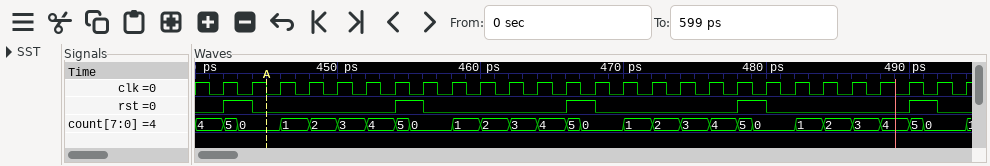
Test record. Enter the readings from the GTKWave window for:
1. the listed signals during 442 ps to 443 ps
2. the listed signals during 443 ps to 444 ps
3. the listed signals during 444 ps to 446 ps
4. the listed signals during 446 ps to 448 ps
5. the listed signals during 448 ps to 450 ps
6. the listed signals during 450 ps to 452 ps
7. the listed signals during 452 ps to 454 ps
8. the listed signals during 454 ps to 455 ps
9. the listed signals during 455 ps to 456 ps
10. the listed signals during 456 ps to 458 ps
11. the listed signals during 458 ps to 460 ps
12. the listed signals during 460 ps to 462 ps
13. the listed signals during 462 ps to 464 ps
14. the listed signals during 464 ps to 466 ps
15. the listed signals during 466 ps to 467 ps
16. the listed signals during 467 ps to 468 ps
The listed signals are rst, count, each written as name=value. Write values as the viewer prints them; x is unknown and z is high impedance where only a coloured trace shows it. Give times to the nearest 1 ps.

rst=1, count=5
rst=1, count=0
rst=0, count=0
rst=0, count=1
rst=0, count=2
rst=0, count=3
rst=0, count=4
rst=1, count=5
rst=1, count=0
rst=0, count=0
rst=0, count=1
rst=0, count=2
rst=0, count=3
rst=0, count=4
rst=1, count=5
rst=1, count=0
